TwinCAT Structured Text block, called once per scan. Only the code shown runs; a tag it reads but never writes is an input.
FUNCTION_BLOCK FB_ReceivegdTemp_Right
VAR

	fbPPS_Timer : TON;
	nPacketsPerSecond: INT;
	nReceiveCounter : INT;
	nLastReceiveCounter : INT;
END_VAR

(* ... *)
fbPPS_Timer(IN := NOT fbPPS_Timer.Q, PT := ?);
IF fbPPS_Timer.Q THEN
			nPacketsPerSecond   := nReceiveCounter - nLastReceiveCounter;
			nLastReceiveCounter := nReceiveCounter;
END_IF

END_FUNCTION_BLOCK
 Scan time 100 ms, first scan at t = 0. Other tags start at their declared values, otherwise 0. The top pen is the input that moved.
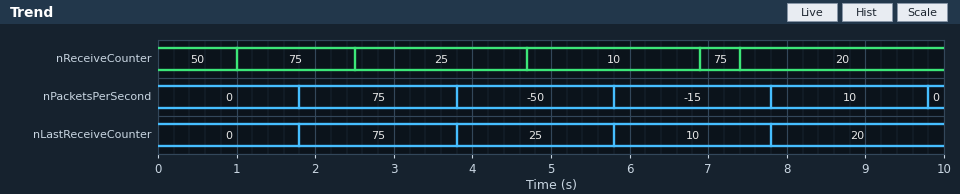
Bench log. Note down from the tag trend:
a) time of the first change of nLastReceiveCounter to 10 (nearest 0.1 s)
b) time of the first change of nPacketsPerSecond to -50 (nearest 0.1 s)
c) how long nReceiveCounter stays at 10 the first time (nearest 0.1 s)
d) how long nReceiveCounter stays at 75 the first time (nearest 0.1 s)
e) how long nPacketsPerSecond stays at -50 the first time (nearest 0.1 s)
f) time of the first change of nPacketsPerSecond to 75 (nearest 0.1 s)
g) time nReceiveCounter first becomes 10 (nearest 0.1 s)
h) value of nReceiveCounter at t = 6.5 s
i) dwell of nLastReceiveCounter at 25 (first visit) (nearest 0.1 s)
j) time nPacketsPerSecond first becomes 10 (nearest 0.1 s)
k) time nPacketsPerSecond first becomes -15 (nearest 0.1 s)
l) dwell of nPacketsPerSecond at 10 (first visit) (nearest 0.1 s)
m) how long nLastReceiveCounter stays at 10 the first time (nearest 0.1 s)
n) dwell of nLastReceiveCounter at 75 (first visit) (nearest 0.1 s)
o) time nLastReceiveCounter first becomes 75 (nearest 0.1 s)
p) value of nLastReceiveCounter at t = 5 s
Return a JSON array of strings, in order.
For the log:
["5.8 s", "3.8 s", "2.2 s", "1.5 s", "2.0 s", "1.8 s", "4.7 s", "10", "2.0 s", "7.8 s", "5.8 s", "2.0 s", "2.0 s", "2.0 s", "1.8 s", "25"]
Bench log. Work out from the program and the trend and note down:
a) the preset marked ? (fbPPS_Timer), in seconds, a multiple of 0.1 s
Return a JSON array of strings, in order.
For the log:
["1.8 s"]
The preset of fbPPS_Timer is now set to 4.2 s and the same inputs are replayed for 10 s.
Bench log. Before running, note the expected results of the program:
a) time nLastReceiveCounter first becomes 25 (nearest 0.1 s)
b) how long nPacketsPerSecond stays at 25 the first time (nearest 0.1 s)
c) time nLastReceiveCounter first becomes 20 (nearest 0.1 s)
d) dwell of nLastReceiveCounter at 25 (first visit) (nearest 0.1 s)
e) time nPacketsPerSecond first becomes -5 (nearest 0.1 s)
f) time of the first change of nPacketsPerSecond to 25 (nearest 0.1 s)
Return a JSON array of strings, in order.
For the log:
["4.2 s", "4.4 s", "8.6 s", "4.4 s", "8.6 s", "4.2 s"]
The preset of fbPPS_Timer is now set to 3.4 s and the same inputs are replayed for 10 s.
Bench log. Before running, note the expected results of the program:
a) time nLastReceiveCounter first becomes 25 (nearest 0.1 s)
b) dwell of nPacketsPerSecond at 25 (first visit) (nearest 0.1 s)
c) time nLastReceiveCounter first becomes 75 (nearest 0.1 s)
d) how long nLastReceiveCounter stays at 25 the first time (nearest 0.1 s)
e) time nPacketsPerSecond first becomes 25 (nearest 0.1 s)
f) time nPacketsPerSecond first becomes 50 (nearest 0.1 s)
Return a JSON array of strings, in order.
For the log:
["3.4 s", "3.6 s", "7.0 s", "3.6 s", "3.4 s", "7.0 s"]
